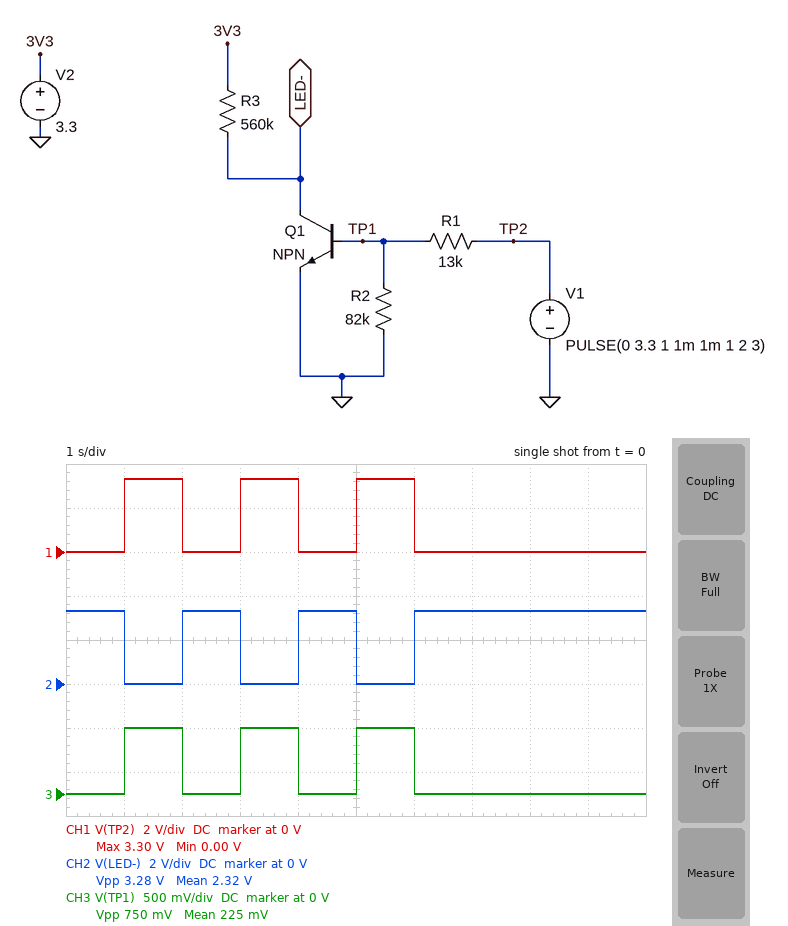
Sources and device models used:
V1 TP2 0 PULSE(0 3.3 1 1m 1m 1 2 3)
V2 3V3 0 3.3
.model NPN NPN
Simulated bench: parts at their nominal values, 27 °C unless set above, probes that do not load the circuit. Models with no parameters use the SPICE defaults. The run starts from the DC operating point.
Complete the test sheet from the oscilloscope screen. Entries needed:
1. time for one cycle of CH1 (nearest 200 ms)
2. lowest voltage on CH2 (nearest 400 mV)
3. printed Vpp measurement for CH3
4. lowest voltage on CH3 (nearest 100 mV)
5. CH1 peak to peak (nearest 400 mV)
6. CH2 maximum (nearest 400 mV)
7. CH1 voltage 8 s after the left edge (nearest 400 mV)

2.0 s
0 V
750 mV
0 V
3.2 V
3.2 V
0 V
